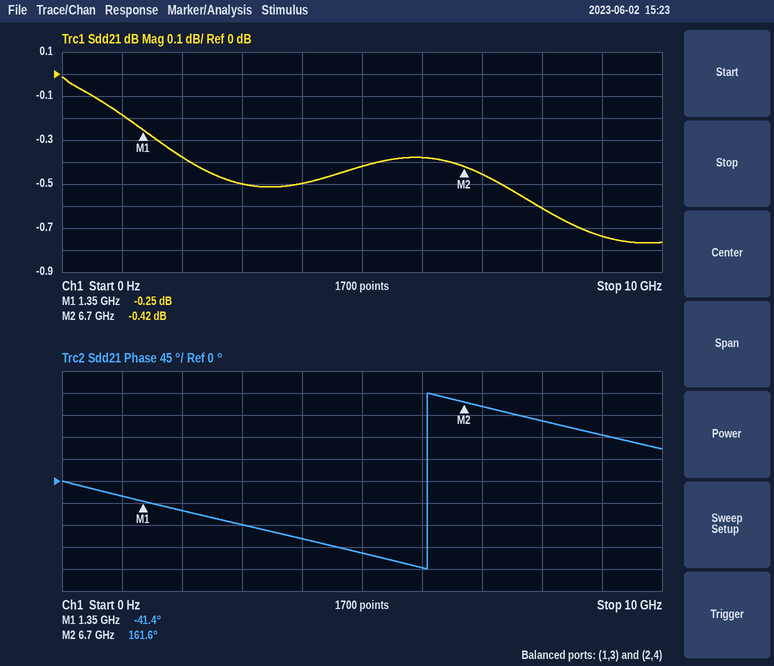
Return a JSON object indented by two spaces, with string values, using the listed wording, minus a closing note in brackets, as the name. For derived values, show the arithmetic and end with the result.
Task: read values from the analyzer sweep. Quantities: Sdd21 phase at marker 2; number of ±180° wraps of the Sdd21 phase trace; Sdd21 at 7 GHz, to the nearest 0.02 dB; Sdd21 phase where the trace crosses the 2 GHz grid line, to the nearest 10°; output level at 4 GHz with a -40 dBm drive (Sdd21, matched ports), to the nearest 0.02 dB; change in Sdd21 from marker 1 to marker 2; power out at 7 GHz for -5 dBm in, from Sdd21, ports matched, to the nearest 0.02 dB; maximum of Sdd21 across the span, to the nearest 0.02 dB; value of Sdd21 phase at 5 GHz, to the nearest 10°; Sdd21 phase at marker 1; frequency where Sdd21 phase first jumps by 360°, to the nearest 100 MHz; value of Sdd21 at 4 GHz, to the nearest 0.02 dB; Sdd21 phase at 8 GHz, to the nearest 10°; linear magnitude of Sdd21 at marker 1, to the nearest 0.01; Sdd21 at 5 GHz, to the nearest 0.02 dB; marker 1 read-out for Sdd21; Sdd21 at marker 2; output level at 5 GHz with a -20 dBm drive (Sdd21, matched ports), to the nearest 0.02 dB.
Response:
{
  "Sdd21 phase at marker 2": "161.6°",
  "number of ±180° wraps of the Sdd21 phase trace": "1",
  "Sdd21 at 7 GHz, to the nearest 0.02 dB": "-0.46 dB",
  "Sdd21 phase where the trace crosses the 2 GHz grid line, to the nearest 10°": "-60°",
  "output level at 4 GHz with a -40 dBm drive (Sdd21, matched ports), to the nearest 0.02 dB": "-40 dBm + (-0.50 dB) = -40.50 dBm",
  "change in Sdd21 from marker 1 to marker 2": "-0.42 − (-0.25) = -0.17 dB",
  "power out at 7 GHz for -5 dBm in, from Sdd21, ports matched, to the nearest 0.02 dB": "-5 dBm + (-0.46 dB) = -5.46 dBm",
  "maximum of Sdd21 across the span, to the nearest 0.02 dB": "-0.02 dB",
  "value of Sdd21 phase at 5 GHz, to the nearest 10°": "-150°",
  "Sdd21 phase at marker 1": "-41.4°",
  "frequency where Sdd21 phase first jumps by 360°, to the nearest 100 MHz": "6.1 GHz",
  "value of Sdd21 at 4 GHz, to the nearest 0.02 dB": "-0.50 dB",
  "Sdd21 phase at 8 GHz, to the nearest 10°": "120°",
  "linear magnitude of Sdd21 at marker 1, to the nearest 0.01": "10^(-0.25/20) ≈ 0.97",
  "Sdd21 at 5 GHz, to the nearest 0.02 dB": "-0.42 dB",
  "marker 1 read-out for Sdd21": "-0.25 dB",
  "Sdd21 at marker 2": "-0.42 dB",
  "output level at 5 GHz with a -20 dBm drive (Sdd21, matched ports), to the nearest 0.02 dB": "-20 dBm + (-0.42 dB) = -20.42 dBm"
}
